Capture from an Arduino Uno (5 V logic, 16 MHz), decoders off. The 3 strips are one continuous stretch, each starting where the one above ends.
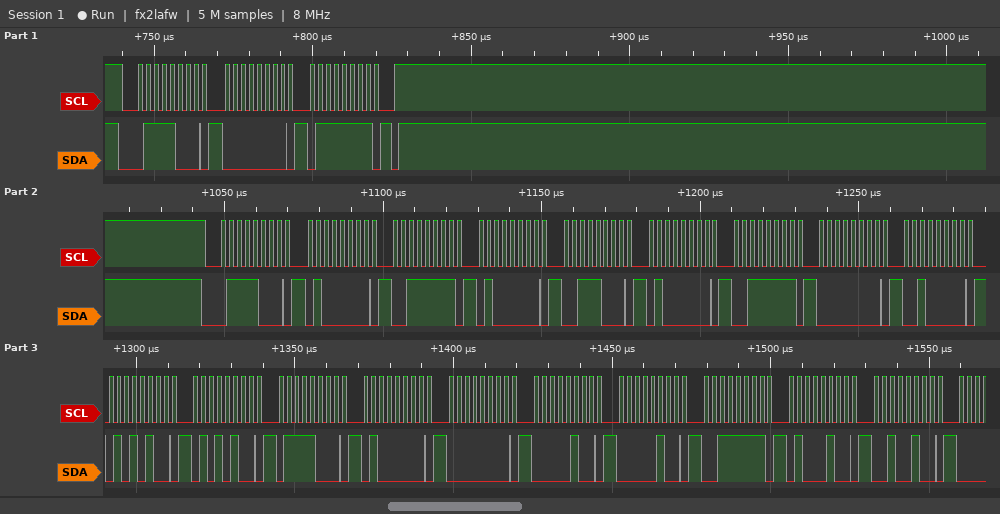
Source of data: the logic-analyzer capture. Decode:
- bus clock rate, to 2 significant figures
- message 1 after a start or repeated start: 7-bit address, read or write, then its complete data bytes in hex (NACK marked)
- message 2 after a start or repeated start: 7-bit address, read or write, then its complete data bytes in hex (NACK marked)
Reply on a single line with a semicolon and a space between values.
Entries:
400 kHz; 0x3C write: 00 7F; 0x3C write: 40 3F 40 38 40 3F 00 20 54 54 78 40 00 04 04 3F 44 24
